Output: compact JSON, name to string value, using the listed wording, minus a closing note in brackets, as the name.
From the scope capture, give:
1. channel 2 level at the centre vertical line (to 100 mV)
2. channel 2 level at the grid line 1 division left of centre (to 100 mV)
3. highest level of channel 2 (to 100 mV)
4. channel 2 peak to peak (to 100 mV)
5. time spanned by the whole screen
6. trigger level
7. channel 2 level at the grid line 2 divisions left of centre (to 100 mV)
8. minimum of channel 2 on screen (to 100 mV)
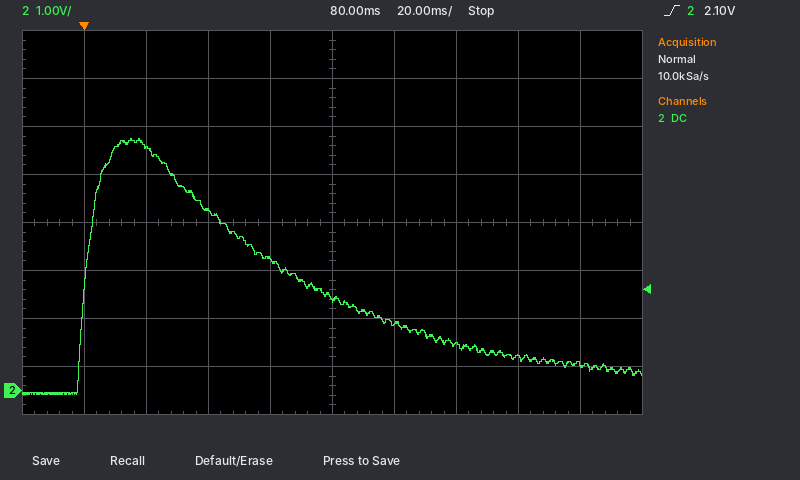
{"channel 2 level at the centre vertical line": "1.9 V", "channel 2 level at the grid line 1 division left of centre": "2.7 V", "highest level of channel 2": "5.2 V", "channel 2 peak to peak": "5.3 V", "time spanned by the whole screen": "200 ms", "trigger level": "2.10 V", "channel 2 level at the grid line 2 divisions left of centre": "3.7 V", "minimum of channel 2 on screen": "-100 mV"}
